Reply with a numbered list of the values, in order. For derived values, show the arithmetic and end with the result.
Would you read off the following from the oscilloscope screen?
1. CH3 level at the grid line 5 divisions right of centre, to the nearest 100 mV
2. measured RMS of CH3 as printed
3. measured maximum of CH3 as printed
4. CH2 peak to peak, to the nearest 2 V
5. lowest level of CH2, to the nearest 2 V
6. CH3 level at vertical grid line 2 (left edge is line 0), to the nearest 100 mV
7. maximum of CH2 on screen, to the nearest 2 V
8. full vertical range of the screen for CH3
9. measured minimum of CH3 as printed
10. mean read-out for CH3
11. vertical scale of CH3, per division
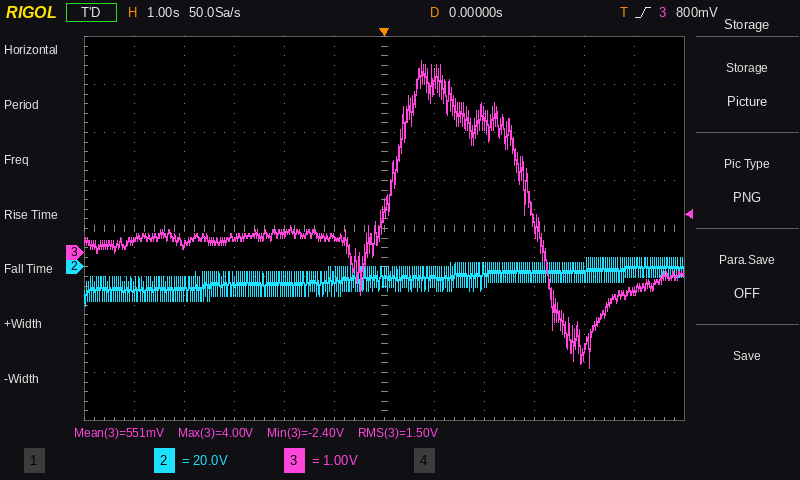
1. -800 mV
2. 1.50 V
3. 4.00 V
4. 4 V − (-16 V) = 20 V
5. -16 V
6. 200 mV
7. 4 V
8. 8 V
9. -2.40 V
10. 551 mV
11. 1 V
